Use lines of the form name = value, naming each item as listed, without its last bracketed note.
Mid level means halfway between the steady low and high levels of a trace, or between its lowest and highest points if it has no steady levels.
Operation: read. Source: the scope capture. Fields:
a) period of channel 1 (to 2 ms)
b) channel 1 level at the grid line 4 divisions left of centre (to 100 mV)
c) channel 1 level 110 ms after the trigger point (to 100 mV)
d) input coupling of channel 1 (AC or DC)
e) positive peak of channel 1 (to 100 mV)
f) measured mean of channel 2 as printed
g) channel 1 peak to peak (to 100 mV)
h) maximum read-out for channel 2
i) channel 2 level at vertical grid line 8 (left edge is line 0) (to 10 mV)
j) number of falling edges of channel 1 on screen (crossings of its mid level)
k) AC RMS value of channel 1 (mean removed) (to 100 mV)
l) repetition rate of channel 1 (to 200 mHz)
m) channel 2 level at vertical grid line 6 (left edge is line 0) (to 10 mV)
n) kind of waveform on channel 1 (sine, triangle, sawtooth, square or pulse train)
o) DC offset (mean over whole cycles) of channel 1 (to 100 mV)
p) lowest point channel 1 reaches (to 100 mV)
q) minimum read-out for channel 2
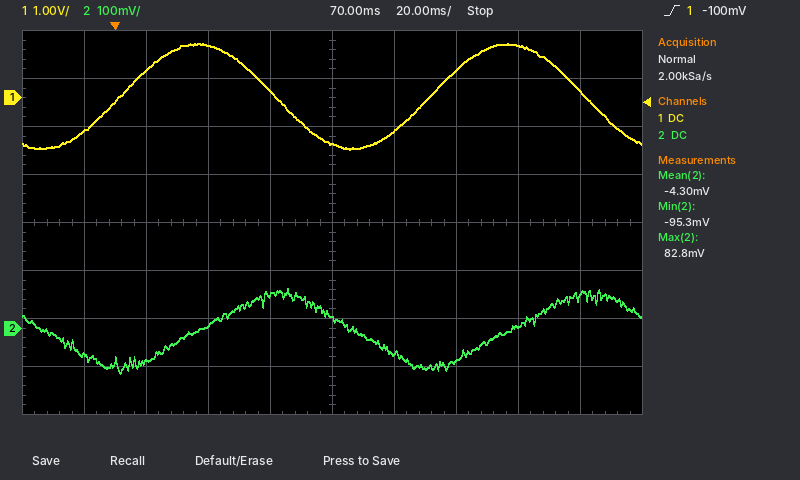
period of channel 1 = 100 ms
channel 1 level at the grid line 4 divisions left of centre = -700 mV
channel 1 level 110 ms after the trigger point = 600 mV
input coupling of channel 1 = DC
positive peak of channel 1 = 1.1 V
measured mean of channel 2 as printed = -4.30 mV
channel 1 peak to peak = 2.2 V
maximum read-out for channel 2 = 82.8 mV
channel 2 level at vertical grid line 8 (left edge is line 0) = 0 mV
number of falling edges of channel 1 on screen = 2
AC RMS value of channel 1 (mean removed) = 800 mV
repetition rate of channel 1 = 10.0 Hz
channel 2 level at vertical grid line 6 (left edge is line 0) = -50 mV
kind of waveform on channel 1 = sine
DC offset (mean over whole cycles) of channel 1 = 0.0 V
lowest point channel 1 reaches = -1.1 V
minimum read-out for channel 2 = -95.3 mV
